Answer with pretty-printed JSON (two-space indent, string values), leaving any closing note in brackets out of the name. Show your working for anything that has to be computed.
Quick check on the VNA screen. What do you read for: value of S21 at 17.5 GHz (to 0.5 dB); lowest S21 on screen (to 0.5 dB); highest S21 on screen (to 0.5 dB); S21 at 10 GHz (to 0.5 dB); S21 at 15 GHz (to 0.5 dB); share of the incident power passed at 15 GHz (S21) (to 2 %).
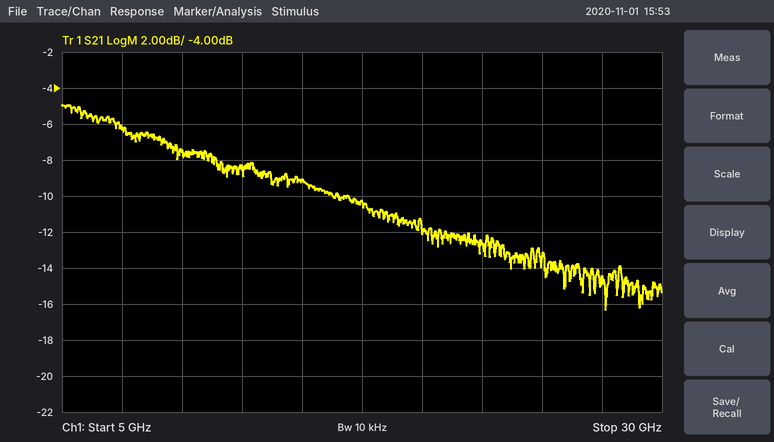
{
  "value of S21 at 17.5 GHz": "-10.5 dB",
  "lowest S21 on screen": "-16.5 dB",
  "highest S21 on screen": "-5.0 dB",
  "S21 at 10 GHz": "-7.5 dB",
  "S21 at 15 GHz": "-9.0 dB",
  "share of the incident power passed at 15 GHz (S21)": "10^(-9/10) ≈ 12.6 %, so 12 % to the nearest 2 %"
}
